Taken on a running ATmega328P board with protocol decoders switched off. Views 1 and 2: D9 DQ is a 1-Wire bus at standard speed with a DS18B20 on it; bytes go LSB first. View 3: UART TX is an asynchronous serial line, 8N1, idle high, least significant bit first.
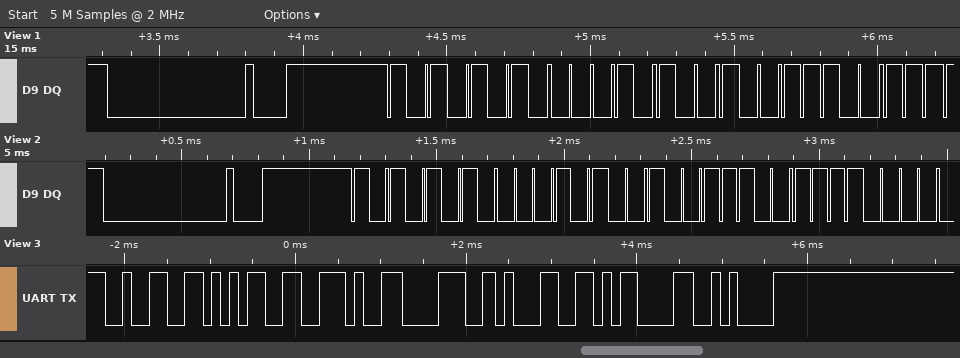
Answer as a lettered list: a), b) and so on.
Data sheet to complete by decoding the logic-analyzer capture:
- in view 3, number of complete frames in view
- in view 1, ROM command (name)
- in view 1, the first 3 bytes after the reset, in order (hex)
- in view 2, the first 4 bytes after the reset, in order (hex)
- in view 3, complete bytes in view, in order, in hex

a) 7
b) Match ROM
c) 55 28 39
d) 55 28 39 0F
e) 32 35 2E 38 31 0D 0A
